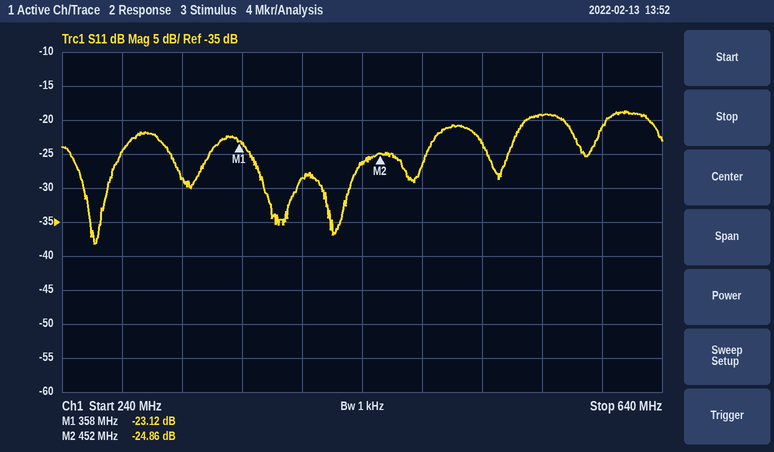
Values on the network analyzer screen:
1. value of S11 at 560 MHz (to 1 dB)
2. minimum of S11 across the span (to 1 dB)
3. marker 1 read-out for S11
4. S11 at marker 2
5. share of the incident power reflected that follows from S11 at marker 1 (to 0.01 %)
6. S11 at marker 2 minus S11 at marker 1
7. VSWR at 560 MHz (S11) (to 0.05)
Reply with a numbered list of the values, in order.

1. -19 dB
2. -38 dB
3. -23.12 dB
4. -24.86 dB
5. 0.49 %
6. -1.74 dB
7. 1.25
